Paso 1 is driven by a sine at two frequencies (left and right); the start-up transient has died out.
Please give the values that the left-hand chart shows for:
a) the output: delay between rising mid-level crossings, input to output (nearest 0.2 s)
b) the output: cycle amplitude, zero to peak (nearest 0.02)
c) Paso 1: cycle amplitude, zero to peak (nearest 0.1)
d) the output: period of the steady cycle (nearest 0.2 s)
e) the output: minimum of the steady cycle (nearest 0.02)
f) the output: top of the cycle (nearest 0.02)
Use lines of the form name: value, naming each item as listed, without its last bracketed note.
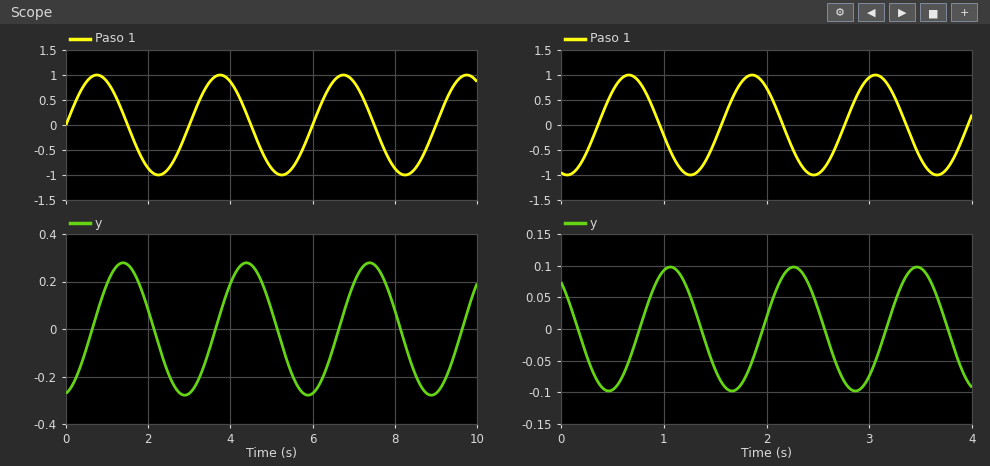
the output: delay between rising mid-level crossings, input to output: 0.6 s
the output: cycle amplitude, zero to peak: 0.28
Paso 1: cycle amplitude, zero to peak: 1.0
the output: period of the steady cycle: 3.0 s
the output: minimum of the steady cycle: -0.28
the output: top of the cycle: 0.28
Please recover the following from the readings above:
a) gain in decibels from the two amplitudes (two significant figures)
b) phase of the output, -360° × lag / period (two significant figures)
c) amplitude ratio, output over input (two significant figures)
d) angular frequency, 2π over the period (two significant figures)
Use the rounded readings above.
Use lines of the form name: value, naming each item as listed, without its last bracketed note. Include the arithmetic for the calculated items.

gain in decibels from the two amplitudes: 20 log10(0.28 / 1) = -11 dB
phase of the output, -360° × lag / period: -360 × 0.6 / 3 = -72°
amplitude ratio, output over input: 0.28 / 1 = 0.28
angular frequency, 2π over the period: 2π / 3 = 2.1 rad/s
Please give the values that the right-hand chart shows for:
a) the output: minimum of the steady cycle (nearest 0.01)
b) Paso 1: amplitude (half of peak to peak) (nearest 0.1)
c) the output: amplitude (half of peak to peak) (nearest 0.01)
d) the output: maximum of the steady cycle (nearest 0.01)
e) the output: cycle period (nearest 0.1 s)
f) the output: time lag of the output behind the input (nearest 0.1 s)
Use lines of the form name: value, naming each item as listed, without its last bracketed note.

the output: minimum of the steady cycle: -0.10
Paso 1: amplitude (half of peak to peak): 1.0
the output: amplitude (half of peak to peak): 0.10
the output: maximum of the steady cycle: 0.10
the output: cycle period: 1.2 s
the output: time lag of the output behind the input: 0.4 s
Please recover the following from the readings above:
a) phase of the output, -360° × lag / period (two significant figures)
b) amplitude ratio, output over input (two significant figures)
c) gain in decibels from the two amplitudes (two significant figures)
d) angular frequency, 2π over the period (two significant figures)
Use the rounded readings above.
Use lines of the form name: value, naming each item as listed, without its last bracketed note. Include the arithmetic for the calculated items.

phase of the output, -360° × lag / period: -360 × 0.4 / 1.2 = -120°
amplitude ratio, output over input: 0.1 / 1 = 0.10
gain in decibels from the two amplitudes: 20 log10(0.1 / 1) = -20 dB
angular frequency, 2π over the period: 2π / 1.2 = 5.2 rad/s
